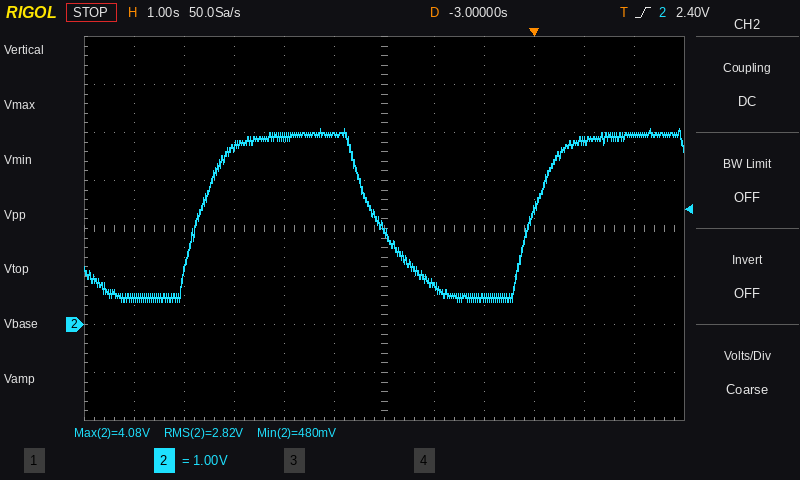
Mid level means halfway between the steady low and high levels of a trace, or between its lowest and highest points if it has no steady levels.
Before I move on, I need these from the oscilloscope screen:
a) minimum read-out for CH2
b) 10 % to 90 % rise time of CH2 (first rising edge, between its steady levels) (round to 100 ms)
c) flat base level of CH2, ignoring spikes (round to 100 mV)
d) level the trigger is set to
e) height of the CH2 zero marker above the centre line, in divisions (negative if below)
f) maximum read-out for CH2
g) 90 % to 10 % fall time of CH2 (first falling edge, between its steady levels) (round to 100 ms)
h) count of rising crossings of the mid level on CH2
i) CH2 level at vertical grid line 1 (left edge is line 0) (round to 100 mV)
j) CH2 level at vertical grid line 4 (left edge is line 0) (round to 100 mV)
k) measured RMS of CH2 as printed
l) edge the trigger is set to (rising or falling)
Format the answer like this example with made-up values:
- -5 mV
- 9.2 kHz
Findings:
- 480 mV
- 900 ms
- 600 mV
- 2.40 V
- -2.0 div
- 4.08 V
- 1.5 s
- 2
- 600 mV
- 3.9 V
- 2.82 V
- rising
